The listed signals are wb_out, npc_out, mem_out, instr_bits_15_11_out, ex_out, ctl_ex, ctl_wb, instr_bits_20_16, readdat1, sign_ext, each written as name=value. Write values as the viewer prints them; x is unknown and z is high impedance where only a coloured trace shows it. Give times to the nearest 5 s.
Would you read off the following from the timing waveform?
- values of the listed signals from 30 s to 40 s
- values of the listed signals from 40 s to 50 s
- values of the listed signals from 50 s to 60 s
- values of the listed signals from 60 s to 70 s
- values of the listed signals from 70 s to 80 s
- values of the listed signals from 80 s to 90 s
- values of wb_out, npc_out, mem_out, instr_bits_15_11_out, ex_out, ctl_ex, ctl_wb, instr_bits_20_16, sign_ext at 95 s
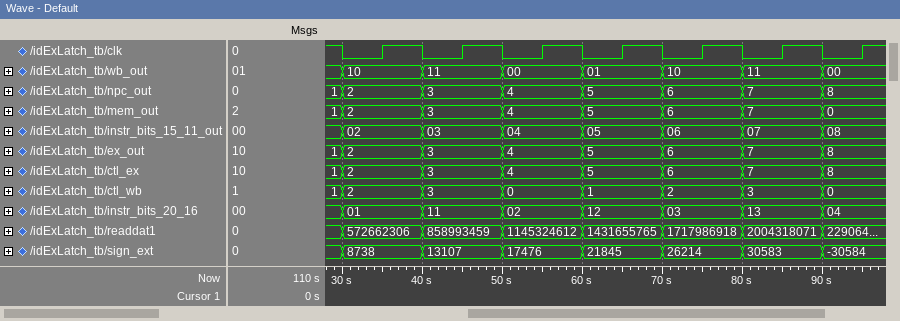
wb_out=10, npc_out=2, mem_out=2, instr_bits_15_11_out=02, ex_out=2, ctl_ex=2, ctl_wb=2, instr_bits_20_16=01, readdat1=572662306, sign_ext=8738
wb_out=11, npc_out=3, mem_out=3, instr_bits_15_11_out=03, ex_out=3, ctl_ex=3, ctl_wb=3, instr_bits_20_16=11, readdat1=858993459, sign_ext=13107
wb_out=00, npc_out=4, mem_out=4, instr_bits_15_11_out=04, ex_out=4, ctl_ex=4, ctl_wb=0, instr_bits_20_16=02, readdat1=1145324612, sign_ext=17476
wb_out=01, npc_out=5, mem_out=5, instr_bits_15_11_out=05, ex_out=5, ctl_ex=5, ctl_wb=1, instr_bits_20_16=12, readdat1=1431655765, sign_ext=21845
wb_out=10, npc_out=6, mem_out=6, instr_bits_15_11_out=06, ex_out=6, ctl_ex=6, ctl_wb=2, instr_bits_20_16=03, readdat1=1717986918, sign_ext=26214
wb_out=11, npc_out=7, mem_out=7, instr_bits_15_11_out=07, ex_out=7, ctl_ex=7, ctl_wb=3, instr_bits_20_16=13, readdat1=2004318071, sign_ext=30583
wb_out=00, npc_out=8, mem_out=0, instr_bits_15_11_out=08, ex_out=8, ctl_ex=8, ctl_wb=0, instr_bits_20_16=04, sign_ext=-30584
